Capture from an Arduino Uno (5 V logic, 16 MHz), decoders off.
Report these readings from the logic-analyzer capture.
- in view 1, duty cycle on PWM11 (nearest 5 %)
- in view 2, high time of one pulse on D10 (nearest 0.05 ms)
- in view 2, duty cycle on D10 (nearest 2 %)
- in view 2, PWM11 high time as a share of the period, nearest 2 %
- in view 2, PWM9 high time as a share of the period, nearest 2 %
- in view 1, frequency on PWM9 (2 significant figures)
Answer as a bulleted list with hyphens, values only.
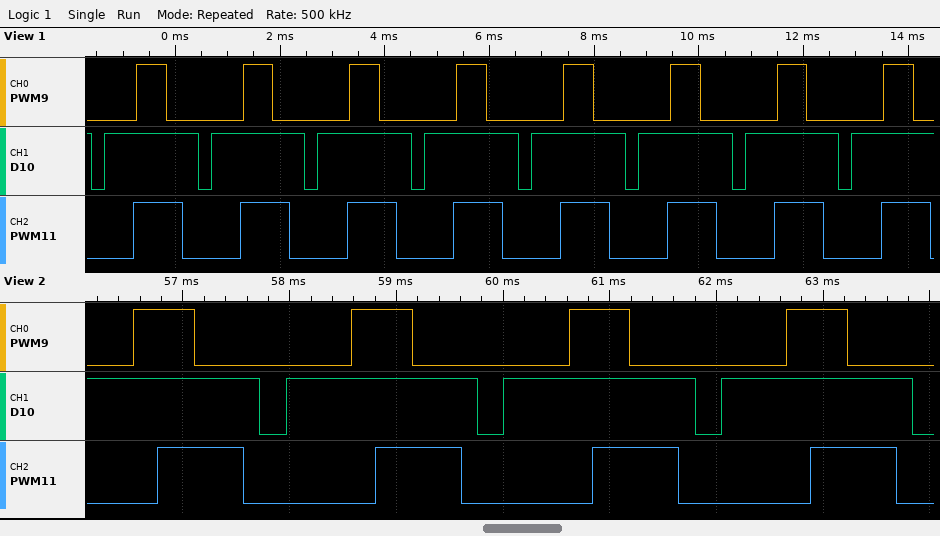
- 45 %
- 1.80 ms
- 88 %
- 40 %
- 28 %
- 490 Hz
